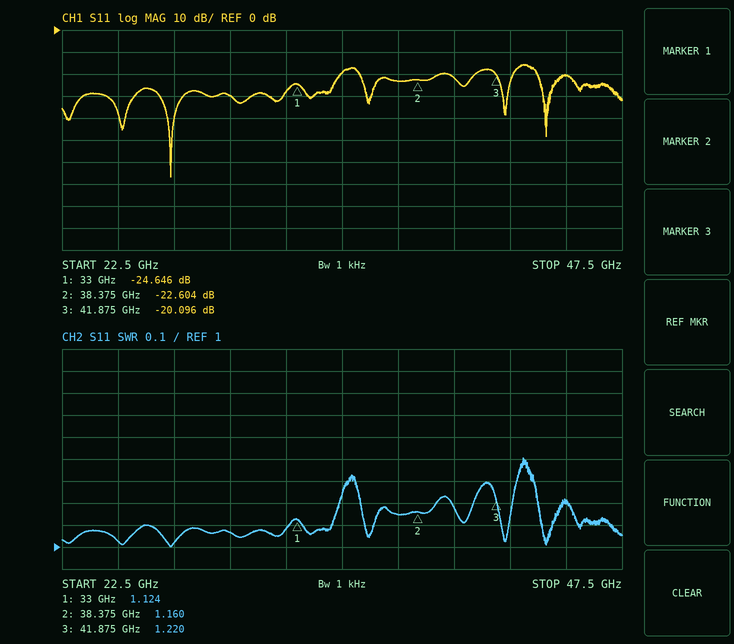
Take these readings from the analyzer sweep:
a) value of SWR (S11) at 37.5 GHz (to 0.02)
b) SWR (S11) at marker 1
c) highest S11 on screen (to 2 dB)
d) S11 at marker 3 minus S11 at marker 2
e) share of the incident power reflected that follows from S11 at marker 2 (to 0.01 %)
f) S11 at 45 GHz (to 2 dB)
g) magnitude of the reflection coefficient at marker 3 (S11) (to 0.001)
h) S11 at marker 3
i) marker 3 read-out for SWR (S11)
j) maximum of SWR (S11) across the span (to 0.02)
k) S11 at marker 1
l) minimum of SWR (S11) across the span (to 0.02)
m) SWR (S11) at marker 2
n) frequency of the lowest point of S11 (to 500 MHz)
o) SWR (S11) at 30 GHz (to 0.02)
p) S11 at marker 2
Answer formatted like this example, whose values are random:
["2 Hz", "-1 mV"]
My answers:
["1.14", "1.124", "-16 dB", "2.508 dB", "0.55 %", "-20 dB", "0.099", "-20.096 dB", "1.220", "1.40", "-24.646 dB", "1.00", "1.160", "27.5 GHz", "1.06", "-22.604 dB"]
